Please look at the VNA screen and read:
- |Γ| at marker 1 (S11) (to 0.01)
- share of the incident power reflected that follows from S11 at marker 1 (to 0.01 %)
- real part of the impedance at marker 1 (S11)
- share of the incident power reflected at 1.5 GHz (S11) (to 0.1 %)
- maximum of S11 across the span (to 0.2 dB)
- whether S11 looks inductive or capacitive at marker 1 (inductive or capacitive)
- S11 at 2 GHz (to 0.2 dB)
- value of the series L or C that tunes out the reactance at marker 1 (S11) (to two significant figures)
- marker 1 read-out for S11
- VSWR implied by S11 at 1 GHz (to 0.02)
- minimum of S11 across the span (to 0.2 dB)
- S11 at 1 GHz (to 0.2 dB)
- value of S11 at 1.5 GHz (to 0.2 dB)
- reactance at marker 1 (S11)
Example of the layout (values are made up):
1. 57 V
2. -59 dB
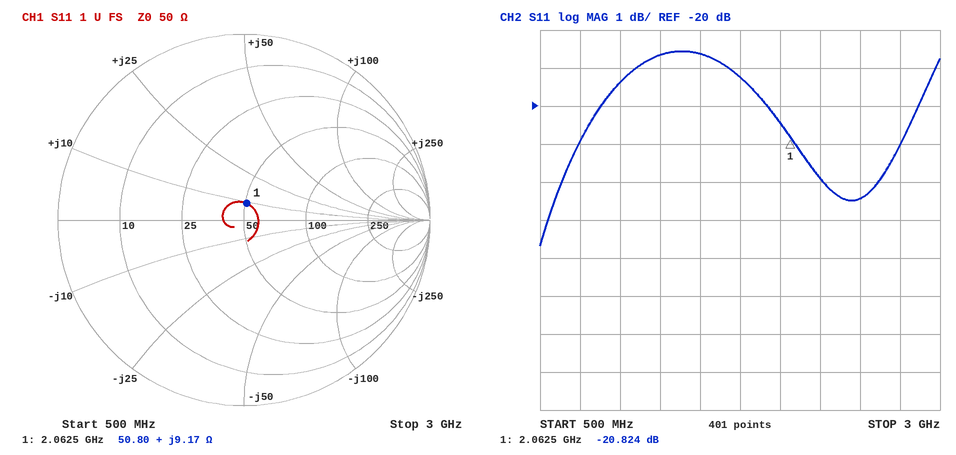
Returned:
1. 0.09
2. 0.83 %
3. 50.80 Ω
4. 1.4 %
5. -18.6 dB
6. inductive
7. -20.4 dB
8. 8.4 pF
9. -20.824 dB
10. 1.24
11. -23.6 dB
12. -19.4 dB
13. -18.6 dB
14. +9.17 Ω
